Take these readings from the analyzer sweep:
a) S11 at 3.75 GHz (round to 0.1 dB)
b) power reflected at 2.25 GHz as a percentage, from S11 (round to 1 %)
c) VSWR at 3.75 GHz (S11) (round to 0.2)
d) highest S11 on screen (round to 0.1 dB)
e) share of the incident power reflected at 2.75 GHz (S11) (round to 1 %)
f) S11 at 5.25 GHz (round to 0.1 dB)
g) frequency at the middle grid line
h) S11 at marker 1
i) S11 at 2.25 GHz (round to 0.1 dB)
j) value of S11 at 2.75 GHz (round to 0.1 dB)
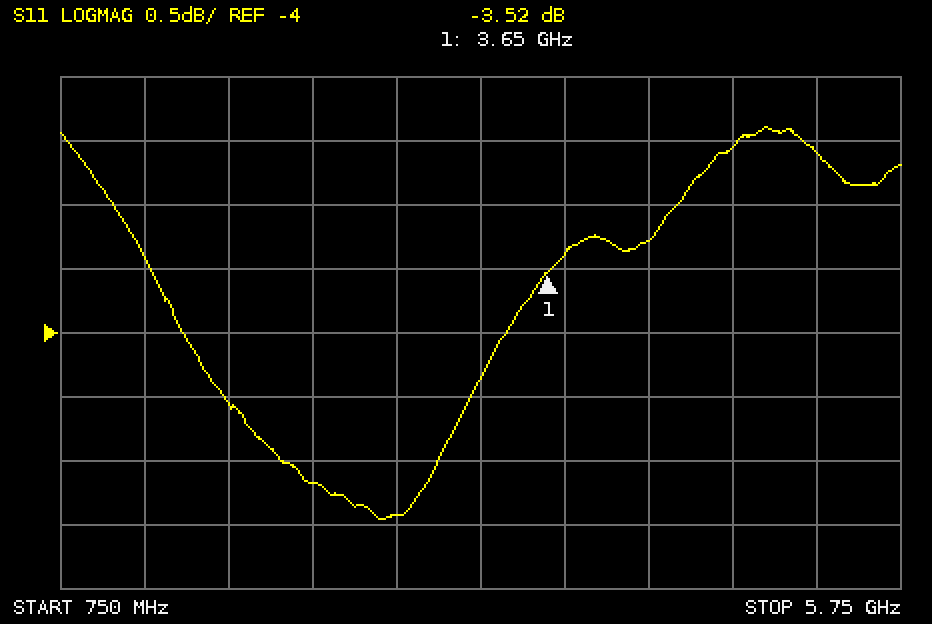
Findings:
-3.4 dB
30 %
5.2
-2.4 dB
29 %
-2.6 dB
3.25 GHz
-3.52 dB
-5.2 dB
-5.4 dB
